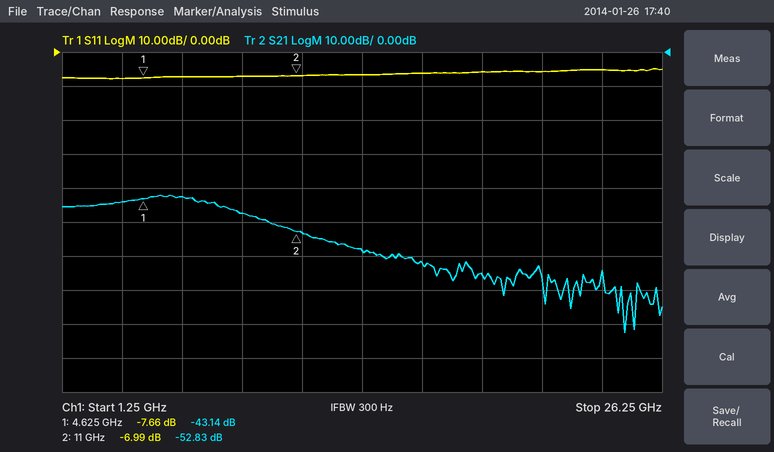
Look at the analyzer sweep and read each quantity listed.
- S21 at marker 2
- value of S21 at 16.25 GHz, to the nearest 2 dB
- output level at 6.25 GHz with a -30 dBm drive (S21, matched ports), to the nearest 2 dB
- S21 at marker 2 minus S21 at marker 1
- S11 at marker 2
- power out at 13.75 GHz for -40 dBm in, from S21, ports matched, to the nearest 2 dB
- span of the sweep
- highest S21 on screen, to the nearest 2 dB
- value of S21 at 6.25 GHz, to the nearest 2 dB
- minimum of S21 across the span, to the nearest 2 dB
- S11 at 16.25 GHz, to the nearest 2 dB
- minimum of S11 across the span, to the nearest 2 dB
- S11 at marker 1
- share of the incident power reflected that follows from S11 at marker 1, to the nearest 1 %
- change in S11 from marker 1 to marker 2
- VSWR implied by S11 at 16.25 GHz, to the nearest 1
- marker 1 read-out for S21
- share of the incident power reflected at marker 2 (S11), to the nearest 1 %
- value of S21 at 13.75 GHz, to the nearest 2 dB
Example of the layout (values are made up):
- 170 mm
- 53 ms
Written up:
- -52.83 dB
- -62 dB
- -72 dBm
- -9.69 dB
- -6.99 dB
- -98 dBm
- 25 GHz
- -42 dB
- -42 dB
- -82 dB
- -6 dB
- -8 dB
- -7.66 dB
- 17 %
- 0.67 dB
- 3
- -43.14 dB
- 20 %
- -58 dB
